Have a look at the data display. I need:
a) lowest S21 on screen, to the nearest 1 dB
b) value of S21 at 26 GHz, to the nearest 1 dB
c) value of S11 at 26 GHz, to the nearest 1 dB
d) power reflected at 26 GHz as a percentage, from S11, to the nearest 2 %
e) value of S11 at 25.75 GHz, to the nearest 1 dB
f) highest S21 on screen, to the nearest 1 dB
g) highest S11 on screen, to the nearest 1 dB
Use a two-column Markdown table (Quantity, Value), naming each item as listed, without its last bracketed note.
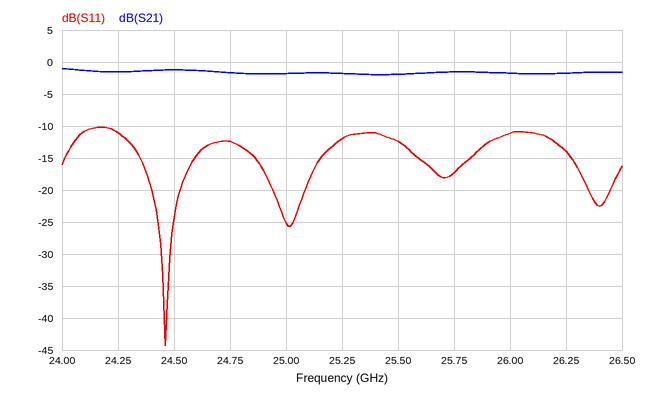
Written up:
| Quantity | Value |
|---|---|
| lowest S21 on screen, to the nearest 1 dB | -2 dB |
| value of S21 at 26 GHz, to the nearest 1 dB | -2 dB |
| value of S11 at 26 GHz, to the nearest 1 dB | -11 dB |
| power reflected at 26 GHz as a percentage, from S11, to the nearest 2 % | 8 % |
| value of S11 at 25.75 GHz, to the nearest 1 dB | -17 dB |
| highest S21 on screen, to the nearest 1 dB | -1 dB |
| highest S11 on screen, to the nearest 1 dB | -10 dB |
